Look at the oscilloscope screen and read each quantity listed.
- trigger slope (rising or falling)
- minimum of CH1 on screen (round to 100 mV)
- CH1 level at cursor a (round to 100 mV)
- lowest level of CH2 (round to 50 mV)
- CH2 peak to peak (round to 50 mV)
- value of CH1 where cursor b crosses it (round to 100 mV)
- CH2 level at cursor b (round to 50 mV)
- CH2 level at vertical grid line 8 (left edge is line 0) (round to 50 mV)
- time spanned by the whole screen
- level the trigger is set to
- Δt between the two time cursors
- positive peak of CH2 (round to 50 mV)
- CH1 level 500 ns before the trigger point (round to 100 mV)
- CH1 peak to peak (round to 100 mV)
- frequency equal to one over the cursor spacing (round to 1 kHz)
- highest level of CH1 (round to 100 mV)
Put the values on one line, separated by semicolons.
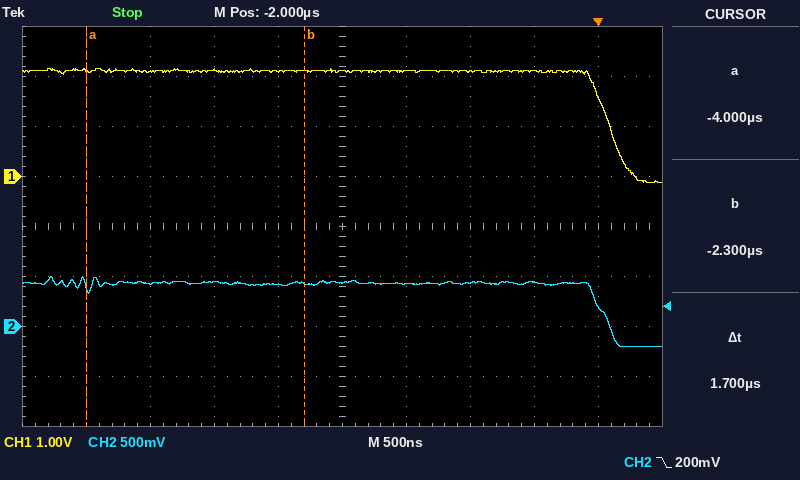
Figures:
falling; -100 mV; 2.1 V; -200 mV; 700 mV; 2.1 V; 450 mV; 450 mV; 5 µs; 200 mV; 1.7 µs; 500 mV; 2.1 V; 2.3 V; 588 kHz; 2.2 V
